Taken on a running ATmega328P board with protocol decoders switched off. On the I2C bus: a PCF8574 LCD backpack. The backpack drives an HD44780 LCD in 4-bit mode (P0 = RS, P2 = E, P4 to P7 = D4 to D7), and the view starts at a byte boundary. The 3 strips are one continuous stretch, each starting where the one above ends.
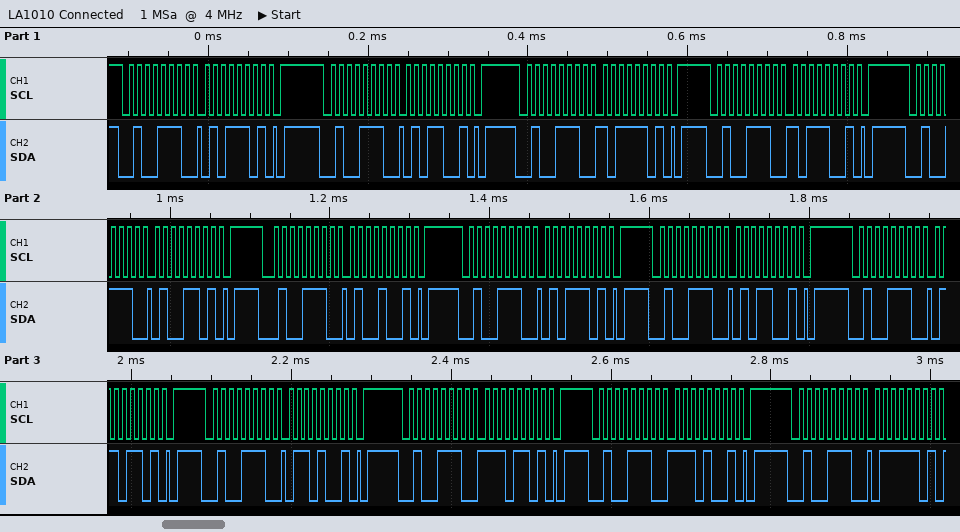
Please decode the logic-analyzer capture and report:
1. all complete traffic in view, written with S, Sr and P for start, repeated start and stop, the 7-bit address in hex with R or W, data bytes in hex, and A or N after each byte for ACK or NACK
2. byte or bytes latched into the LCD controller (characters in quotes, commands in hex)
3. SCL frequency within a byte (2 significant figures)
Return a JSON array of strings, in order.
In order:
["S 27W A 5D A P S 27W A 59 A P S 27W A BD A P S 27W A B9 A P S 27W A 4D A P S 27W A 49 A P S 27W A 5D A P S 27W A 59 A P S 27W A 6D A P S 27W A 69 A P S 27W A ED A P S 27W A E9 A P S 27W A 7D A", "'[' 'E' 'n'", "100 kHz"]
